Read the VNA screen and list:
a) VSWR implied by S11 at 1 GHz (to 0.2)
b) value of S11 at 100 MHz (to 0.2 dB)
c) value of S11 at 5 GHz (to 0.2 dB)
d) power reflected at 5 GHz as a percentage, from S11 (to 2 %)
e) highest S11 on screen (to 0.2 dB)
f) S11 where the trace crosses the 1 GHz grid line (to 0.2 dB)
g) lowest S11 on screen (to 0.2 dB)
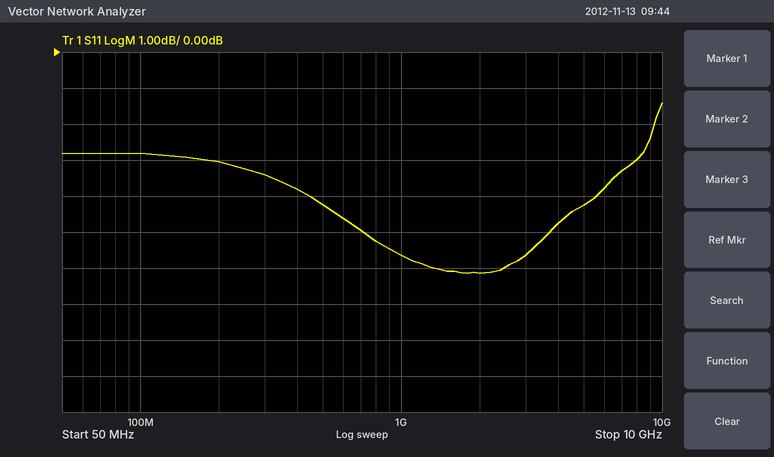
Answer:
3.2
-2.8 dB
-4.2 dB
38 %
-1.4 dB
-5.6 dB
-6.2 dB
